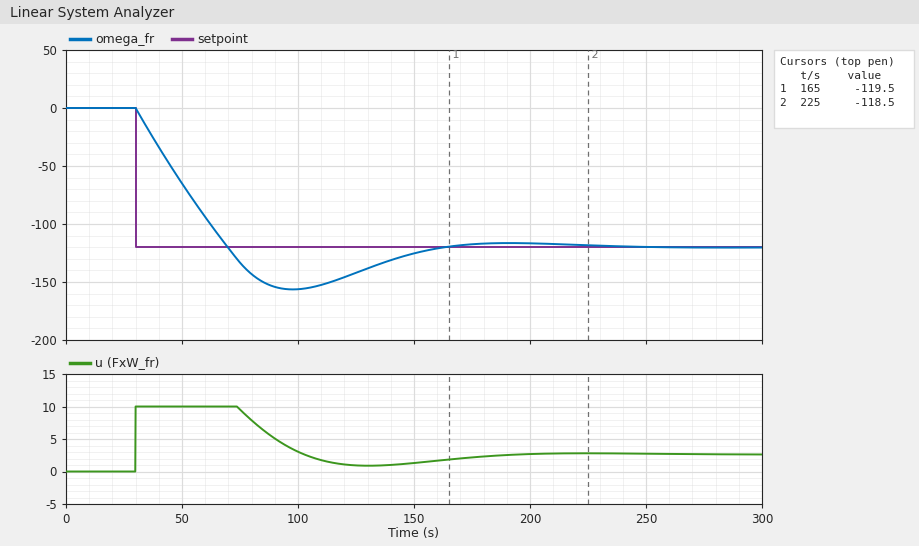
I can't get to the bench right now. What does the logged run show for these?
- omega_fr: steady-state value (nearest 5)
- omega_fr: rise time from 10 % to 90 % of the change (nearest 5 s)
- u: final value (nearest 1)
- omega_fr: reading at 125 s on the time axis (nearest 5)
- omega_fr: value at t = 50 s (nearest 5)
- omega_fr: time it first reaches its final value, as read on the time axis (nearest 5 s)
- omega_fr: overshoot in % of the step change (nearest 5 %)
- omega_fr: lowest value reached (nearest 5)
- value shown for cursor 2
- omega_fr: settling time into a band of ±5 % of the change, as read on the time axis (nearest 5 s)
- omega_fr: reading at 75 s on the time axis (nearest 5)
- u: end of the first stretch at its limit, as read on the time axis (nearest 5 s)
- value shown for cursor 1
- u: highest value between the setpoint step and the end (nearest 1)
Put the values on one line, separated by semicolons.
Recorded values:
-120; 30 s; 3; -140; -65; 70 s; 30 %; -155; -118.5; 150 s; -135; 75 s; -119.5; 10
